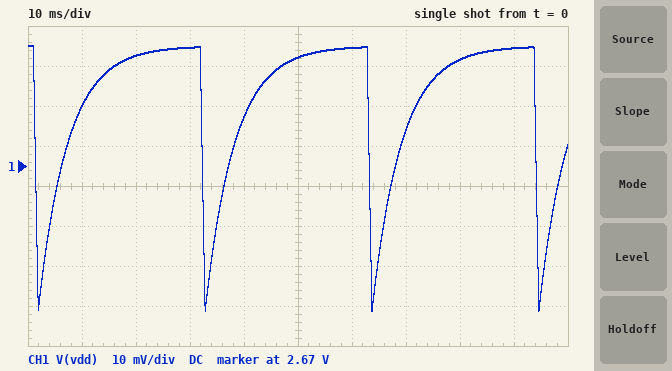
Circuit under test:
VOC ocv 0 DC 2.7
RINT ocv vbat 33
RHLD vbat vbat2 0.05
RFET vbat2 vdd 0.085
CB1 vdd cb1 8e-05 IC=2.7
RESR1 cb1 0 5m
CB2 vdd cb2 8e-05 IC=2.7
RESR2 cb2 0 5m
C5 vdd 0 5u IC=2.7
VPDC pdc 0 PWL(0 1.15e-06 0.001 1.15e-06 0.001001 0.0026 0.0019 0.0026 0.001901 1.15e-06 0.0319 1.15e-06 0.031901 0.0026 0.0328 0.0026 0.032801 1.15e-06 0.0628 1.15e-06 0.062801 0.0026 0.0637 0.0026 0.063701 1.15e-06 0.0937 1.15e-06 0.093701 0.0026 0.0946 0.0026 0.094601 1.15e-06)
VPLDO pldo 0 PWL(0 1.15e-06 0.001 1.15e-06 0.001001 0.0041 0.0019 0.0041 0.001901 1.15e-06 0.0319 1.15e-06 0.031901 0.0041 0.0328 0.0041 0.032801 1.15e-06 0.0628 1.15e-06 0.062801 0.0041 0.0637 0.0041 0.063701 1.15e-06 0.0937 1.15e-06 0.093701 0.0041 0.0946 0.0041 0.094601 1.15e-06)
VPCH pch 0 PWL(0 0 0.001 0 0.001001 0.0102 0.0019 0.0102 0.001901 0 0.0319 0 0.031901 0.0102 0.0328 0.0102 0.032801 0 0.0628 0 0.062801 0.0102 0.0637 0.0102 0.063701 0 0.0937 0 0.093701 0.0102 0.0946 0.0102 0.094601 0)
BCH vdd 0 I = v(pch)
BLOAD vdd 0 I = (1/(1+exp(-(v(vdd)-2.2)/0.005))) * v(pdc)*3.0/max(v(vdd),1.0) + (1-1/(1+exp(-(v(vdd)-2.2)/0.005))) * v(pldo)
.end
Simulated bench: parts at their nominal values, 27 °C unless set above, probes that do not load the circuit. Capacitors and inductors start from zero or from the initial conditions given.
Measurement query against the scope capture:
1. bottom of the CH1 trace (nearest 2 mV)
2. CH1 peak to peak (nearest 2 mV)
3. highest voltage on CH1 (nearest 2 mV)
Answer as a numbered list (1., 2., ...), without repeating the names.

1. 2.634 V
2. 66 mV
3. 2.700 V
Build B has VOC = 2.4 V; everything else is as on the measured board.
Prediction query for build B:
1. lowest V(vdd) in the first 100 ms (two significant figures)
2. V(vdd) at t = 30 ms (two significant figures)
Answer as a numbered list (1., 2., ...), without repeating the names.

1. 2.3 V
2. 2.4 V
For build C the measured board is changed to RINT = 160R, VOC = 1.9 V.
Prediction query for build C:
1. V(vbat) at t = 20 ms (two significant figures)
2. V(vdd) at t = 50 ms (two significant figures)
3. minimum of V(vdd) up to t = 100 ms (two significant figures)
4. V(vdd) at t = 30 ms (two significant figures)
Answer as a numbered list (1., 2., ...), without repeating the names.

1. 2.2 V
2. 2.0 V
3. 1.8 V
4. 2.1 V
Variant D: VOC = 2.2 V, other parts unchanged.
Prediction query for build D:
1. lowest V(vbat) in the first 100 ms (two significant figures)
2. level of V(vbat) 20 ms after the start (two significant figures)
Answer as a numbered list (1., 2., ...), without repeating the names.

1. 2.1 V
2. 2.2 V
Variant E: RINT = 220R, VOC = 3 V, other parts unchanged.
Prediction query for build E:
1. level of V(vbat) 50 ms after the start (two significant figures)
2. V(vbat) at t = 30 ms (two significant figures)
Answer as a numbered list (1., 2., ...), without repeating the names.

1. 2.9 V
2. 2.8 V
